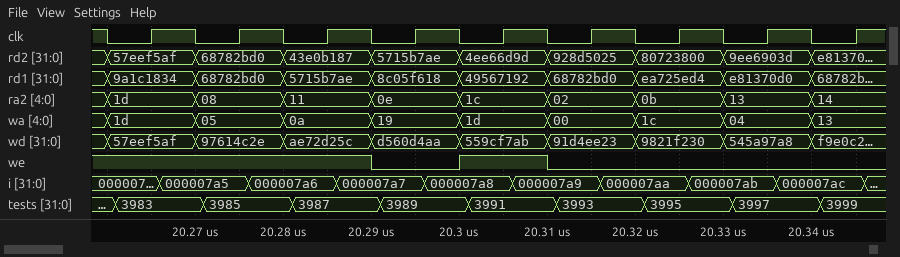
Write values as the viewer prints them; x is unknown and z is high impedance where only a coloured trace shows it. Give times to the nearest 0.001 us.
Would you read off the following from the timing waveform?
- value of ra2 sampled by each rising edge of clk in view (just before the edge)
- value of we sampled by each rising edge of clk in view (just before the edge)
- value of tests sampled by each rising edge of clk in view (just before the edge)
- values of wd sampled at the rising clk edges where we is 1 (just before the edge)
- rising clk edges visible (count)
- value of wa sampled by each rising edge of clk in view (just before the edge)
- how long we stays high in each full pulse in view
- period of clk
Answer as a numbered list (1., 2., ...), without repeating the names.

1. 1d, 08, 11, 0e, 1c, 02, 0b, 13, 14
2. 1 1 1 0 1 0 0 0 0
3. 3983, 3985, 3987, 3989, 3991, 3993, 3995, 3997, 3999
4. 57eef5af, 97614c2e, ae72d25c, 559cf7ab
5. 9
6. 1d, 05, 0a, 19, 1d, 00, 1c, 04, 13
7. 0.01 us
8. 0.01 us
